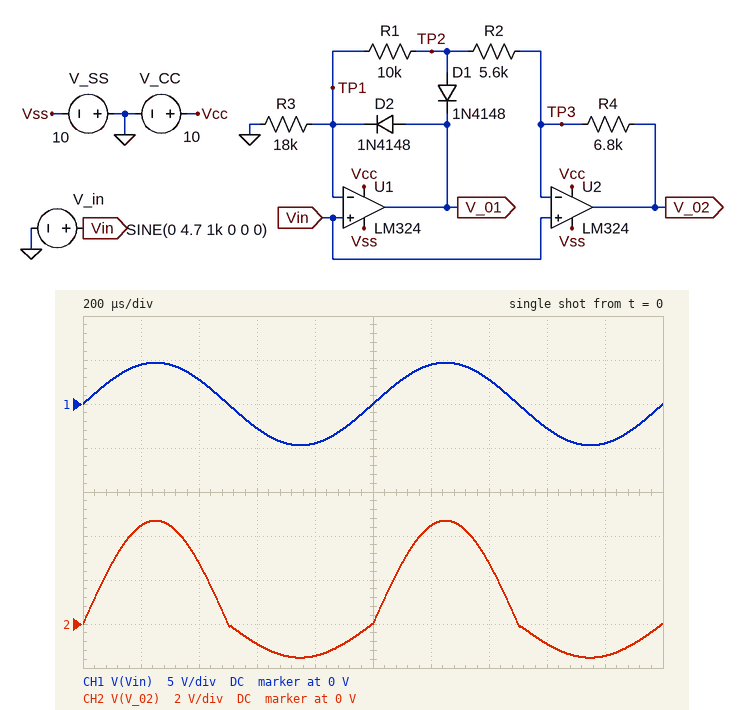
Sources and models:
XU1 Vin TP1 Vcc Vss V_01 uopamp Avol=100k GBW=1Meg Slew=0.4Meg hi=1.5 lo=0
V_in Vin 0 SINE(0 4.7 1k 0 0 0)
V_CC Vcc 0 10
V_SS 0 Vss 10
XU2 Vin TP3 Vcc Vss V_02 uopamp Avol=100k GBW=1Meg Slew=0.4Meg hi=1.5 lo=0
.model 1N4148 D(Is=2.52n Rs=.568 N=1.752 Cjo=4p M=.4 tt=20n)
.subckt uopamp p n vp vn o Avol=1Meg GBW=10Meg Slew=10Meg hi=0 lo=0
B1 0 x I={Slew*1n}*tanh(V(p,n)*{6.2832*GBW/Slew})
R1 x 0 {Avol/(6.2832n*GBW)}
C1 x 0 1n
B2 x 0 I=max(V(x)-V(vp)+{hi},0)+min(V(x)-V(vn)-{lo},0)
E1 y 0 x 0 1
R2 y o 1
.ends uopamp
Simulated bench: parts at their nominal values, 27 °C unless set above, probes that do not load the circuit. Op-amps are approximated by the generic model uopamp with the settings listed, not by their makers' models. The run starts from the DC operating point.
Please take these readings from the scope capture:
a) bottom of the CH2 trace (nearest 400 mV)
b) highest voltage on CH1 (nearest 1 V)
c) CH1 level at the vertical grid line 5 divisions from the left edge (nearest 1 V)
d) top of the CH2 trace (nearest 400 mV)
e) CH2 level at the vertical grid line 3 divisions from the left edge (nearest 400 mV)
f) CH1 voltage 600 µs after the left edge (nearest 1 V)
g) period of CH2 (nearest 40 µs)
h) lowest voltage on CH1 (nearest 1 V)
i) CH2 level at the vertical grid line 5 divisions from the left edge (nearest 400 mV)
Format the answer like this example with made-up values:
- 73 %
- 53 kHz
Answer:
- -1.6 V
- 5 V
- 0 V
- 4.8 V
- -800 mV
- -3 V
- 1.00 ms
- -5 V
- 0 V
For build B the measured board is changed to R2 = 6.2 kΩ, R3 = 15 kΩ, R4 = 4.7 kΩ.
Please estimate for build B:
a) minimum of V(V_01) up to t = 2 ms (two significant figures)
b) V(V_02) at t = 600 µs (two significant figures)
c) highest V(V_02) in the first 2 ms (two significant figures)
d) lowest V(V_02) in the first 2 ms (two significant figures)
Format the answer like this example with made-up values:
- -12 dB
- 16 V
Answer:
- -8.4 V
- -1.4 V
- 4.7 V
- -2.3 V
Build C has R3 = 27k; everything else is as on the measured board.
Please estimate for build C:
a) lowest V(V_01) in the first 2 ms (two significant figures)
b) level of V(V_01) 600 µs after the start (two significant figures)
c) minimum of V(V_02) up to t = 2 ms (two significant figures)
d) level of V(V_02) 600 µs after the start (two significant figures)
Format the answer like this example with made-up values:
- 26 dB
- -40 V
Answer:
- -7.0 V
- -4.3 V
- -2.6 V
- -1.5 V
